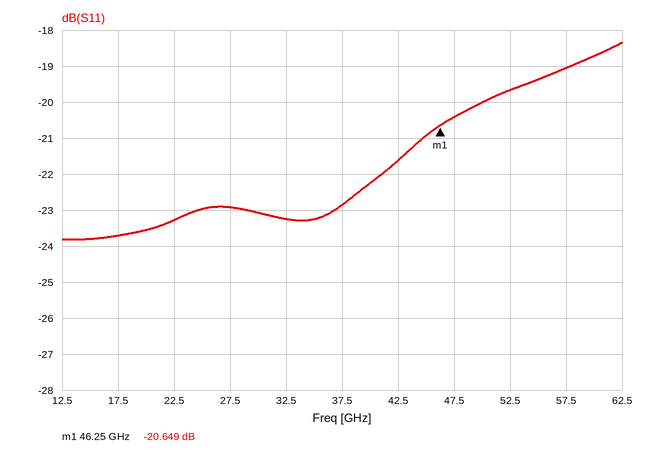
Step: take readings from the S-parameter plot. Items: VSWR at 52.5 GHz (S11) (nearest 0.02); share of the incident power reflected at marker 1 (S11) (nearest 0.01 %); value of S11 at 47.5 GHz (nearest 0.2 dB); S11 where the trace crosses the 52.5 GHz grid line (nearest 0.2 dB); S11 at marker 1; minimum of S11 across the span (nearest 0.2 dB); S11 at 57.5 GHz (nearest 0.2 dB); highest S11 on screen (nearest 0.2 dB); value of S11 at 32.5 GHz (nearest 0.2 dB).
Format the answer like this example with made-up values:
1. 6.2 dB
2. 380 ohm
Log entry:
1. 1.24
2. 0.86 %
3. -20.4 dB
4. -19.6 dB
5. -20.649 dB
6. -23.8 dB
7. -19.0 dB
8. -18.4 dB
9. -23.2 dB
